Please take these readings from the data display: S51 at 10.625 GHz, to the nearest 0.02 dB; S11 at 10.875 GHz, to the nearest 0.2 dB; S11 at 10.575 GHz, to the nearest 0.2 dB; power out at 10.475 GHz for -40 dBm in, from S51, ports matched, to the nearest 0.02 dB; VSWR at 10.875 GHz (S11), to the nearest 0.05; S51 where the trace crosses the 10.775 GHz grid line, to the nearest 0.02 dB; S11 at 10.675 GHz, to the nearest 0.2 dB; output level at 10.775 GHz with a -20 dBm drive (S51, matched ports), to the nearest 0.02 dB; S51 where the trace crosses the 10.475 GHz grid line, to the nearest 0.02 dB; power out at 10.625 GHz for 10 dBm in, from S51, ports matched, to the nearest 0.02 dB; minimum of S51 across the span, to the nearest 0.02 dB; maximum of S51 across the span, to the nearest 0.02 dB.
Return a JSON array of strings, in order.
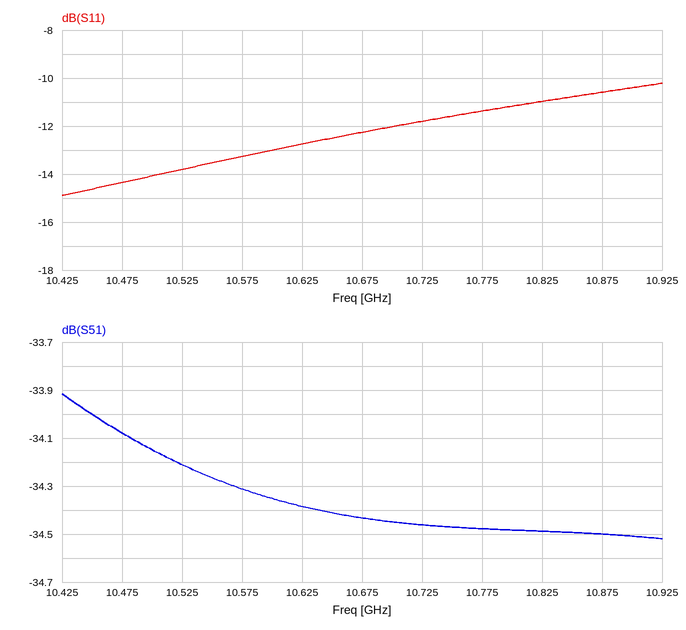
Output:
["-34.38 dB", "-10.6 dB", "-13.2 dB", "-74.08 dBm", "1.85", "-34.48 dB", "-12.2 dB", "-54.48 dBm", "-34.08 dB", "-24.38 dBm", "-34.52 dB", "-33.92 dB"]
